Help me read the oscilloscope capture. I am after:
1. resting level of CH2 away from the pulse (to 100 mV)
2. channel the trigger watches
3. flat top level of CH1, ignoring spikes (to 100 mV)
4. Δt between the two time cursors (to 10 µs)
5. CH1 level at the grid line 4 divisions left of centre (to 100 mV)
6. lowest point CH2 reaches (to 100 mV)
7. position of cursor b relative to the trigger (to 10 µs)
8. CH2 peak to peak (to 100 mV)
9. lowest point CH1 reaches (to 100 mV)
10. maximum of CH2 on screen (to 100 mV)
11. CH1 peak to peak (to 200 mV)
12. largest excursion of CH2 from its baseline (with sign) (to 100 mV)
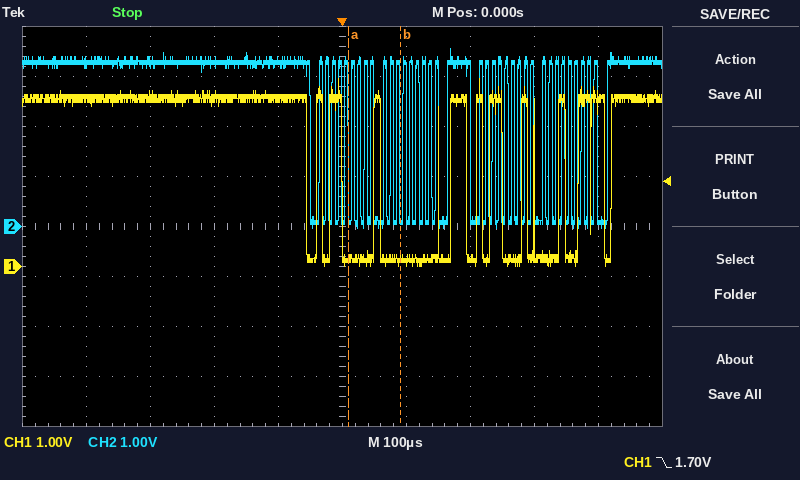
3.3 V
CH1
3.4 V
80 µs
3.4 V
0.0 V
+90 µs
3.6 V
0.0 V
3.6 V
3.8 V
-3.3 V
